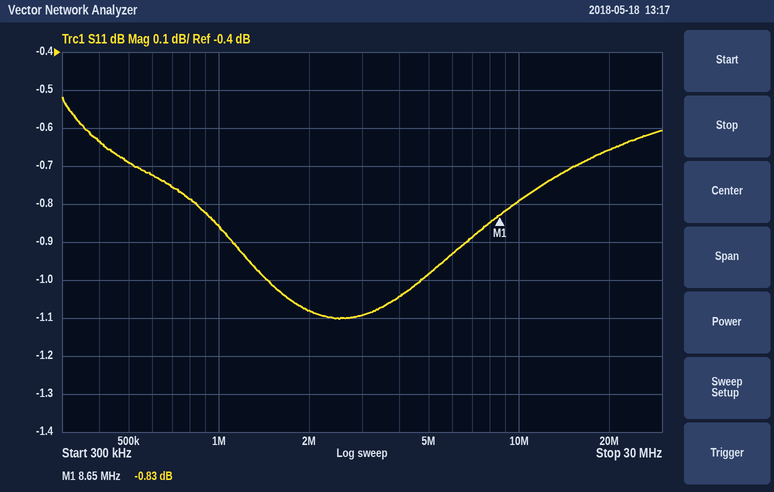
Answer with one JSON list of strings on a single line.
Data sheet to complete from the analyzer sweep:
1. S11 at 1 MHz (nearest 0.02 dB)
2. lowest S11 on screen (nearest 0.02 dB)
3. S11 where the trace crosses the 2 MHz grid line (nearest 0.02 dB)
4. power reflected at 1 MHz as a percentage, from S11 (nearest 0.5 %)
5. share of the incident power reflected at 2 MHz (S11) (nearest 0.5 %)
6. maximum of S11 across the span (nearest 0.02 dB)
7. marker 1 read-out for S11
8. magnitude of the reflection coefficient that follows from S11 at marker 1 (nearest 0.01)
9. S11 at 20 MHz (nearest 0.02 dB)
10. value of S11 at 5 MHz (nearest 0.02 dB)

["-0.86 dB", "-1.10 dB", "-1.08 dB", "82.0 %", "78.0 %", "-0.52 dB", "-0.83 dB", "0.91", "-0.66 dB", "-0.98 dB"]
